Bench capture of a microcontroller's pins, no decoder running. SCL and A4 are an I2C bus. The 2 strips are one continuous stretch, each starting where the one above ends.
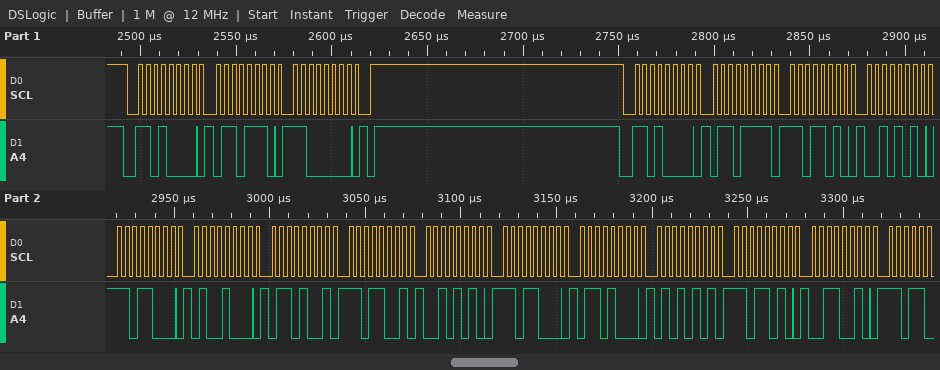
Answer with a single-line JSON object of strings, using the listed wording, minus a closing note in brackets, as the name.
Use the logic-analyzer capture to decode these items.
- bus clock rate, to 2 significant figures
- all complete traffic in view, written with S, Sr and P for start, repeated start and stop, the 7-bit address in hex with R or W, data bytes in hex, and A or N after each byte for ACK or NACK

{"bus clock rate, to 2 significant figures": "250 kHz", "all complete traffic in view, written with S, Sr and P for start, repeated start and stop, the 7-bit address in hex with R or W, data bytes in hex, and A or N after each byte for ACK or NACK": "S 68W A 6E A C0 A P S 68W A 6F A DA A 2A A D8 A 48 A 69 A D9 A 2A A D8 A 68 A 55 A DA A 32 A"}
